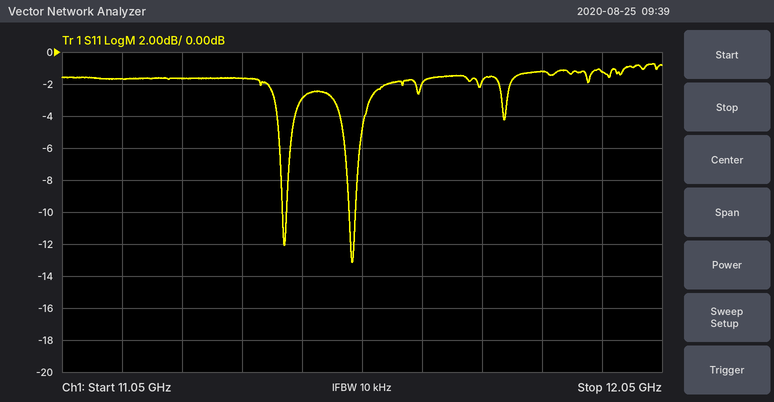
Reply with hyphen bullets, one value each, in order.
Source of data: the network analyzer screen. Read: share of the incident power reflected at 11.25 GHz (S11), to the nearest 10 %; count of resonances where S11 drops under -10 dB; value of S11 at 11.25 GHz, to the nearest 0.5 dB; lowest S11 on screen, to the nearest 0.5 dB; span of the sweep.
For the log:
- 70 %
- 2
- -1.5 dB
- -13.0 dB
- 1 GHz
